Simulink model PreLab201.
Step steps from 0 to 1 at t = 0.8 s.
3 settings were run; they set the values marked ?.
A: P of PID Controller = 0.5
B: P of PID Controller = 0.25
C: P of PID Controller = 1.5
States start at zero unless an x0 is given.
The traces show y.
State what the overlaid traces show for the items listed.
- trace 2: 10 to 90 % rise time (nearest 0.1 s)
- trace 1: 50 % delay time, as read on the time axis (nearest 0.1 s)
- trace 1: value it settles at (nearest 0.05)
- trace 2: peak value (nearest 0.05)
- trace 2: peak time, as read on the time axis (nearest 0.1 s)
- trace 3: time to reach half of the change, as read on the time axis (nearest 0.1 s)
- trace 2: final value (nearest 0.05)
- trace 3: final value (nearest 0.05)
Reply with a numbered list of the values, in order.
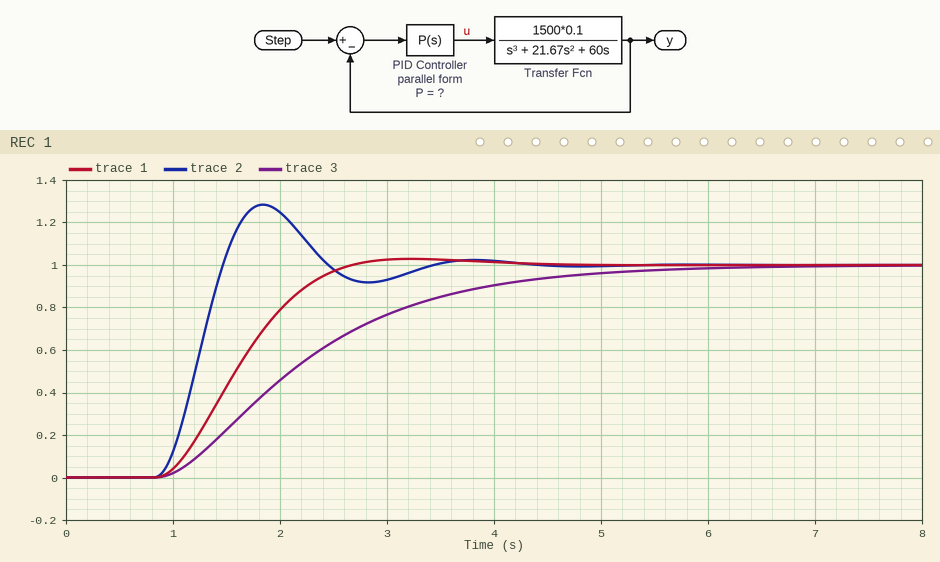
1. 0.4 s
2. 1.6 s
3. 1.00
4. 1.30
5. 1.8 s
6. 2.1 s
7. 1.00
8. 1.00
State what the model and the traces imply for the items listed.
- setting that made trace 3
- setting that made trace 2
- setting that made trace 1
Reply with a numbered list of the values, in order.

1. B
2. C
3. A
